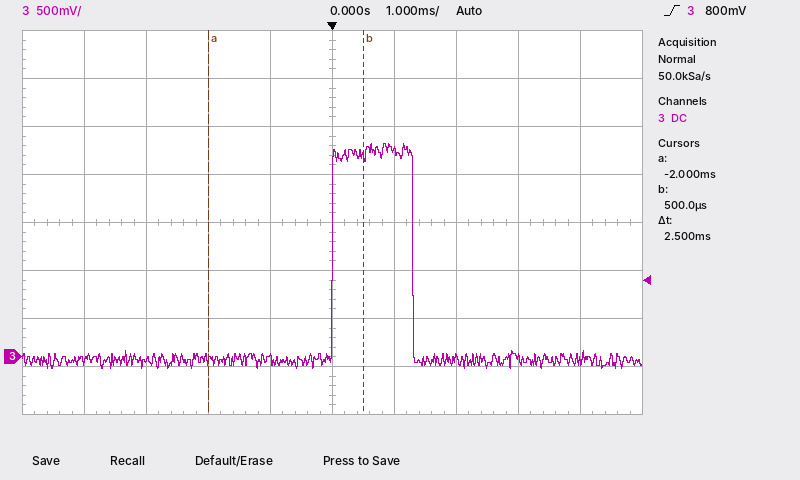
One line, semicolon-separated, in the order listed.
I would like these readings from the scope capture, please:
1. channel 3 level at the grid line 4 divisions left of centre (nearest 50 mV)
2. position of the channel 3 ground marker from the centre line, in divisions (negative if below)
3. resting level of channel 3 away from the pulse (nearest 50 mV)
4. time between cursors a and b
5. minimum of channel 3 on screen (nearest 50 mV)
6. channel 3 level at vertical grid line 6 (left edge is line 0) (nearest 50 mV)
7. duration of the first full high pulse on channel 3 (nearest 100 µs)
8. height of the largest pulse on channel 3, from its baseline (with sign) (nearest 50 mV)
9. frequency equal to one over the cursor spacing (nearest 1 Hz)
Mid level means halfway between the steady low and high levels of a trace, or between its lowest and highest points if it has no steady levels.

-50 mV; -2.8 div; -50 mV; 2.5 ms; -100 mV; 2.15 V; 1.3 ms; +2.25 V; 400 Hz
